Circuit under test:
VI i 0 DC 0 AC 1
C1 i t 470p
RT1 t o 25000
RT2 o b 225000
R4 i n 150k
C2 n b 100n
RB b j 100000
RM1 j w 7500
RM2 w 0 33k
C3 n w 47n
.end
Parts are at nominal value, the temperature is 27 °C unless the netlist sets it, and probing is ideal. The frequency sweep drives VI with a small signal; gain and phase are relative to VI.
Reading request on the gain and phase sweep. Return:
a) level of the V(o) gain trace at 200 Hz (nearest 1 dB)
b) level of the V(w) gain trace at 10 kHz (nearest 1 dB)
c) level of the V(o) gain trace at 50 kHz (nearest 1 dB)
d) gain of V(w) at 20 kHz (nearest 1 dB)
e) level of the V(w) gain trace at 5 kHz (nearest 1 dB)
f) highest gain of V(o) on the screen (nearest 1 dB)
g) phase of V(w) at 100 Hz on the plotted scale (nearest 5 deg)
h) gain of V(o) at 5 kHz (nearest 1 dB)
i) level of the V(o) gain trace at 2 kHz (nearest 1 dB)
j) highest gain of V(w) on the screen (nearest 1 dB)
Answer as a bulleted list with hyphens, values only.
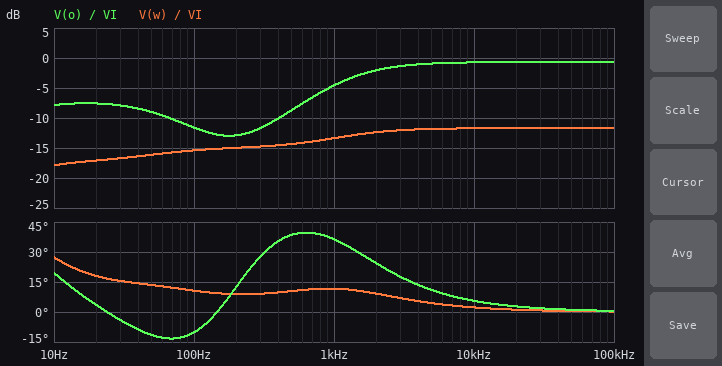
- -13 dB
- -12 dB
- -1 dB
- -12 dB
- -12 dB
- -1 dB
- 10 deg
- -1 dB
- -2 dB
- -12 dB
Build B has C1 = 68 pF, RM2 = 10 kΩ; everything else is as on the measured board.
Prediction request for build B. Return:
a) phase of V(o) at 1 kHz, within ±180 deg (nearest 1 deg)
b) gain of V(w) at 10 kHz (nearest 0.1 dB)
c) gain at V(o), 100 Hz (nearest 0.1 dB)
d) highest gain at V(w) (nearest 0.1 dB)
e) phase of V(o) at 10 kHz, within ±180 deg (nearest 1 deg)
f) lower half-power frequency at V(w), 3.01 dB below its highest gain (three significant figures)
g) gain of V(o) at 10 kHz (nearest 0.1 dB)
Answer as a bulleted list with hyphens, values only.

- 45 deg
- -21.6 dB
- -13.8 dB
- -20.3 dB
- 38 deg
- 3.63 kHz
- -3.4 dB
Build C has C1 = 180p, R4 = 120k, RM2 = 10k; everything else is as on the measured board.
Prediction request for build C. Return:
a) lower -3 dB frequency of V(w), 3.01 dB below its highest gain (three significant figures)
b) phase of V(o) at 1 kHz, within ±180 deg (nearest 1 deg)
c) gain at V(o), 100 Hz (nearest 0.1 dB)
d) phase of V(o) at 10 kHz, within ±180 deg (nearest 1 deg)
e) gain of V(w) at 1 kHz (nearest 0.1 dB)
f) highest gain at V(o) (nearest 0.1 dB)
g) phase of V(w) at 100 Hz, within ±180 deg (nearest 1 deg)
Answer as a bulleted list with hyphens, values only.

- 605 Hz
- 55 deg
- -12.4 dB
- 17 deg
- -22.0 dB
- -0.8 dB
- 13 deg
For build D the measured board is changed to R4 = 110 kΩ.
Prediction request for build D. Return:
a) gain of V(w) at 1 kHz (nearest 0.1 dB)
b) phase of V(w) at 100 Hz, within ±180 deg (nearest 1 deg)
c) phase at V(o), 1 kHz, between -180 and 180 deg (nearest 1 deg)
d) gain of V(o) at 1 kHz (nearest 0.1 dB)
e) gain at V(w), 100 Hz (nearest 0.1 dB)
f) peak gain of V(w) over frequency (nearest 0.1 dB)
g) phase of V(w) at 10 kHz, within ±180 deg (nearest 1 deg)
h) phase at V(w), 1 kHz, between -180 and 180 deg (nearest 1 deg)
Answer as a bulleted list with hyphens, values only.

- -11.7 dB
- 12 deg
- 33 deg
- -4.4 dB
- -13.4 dB
- -10.4 dB
- 2 deg
- 9 deg
